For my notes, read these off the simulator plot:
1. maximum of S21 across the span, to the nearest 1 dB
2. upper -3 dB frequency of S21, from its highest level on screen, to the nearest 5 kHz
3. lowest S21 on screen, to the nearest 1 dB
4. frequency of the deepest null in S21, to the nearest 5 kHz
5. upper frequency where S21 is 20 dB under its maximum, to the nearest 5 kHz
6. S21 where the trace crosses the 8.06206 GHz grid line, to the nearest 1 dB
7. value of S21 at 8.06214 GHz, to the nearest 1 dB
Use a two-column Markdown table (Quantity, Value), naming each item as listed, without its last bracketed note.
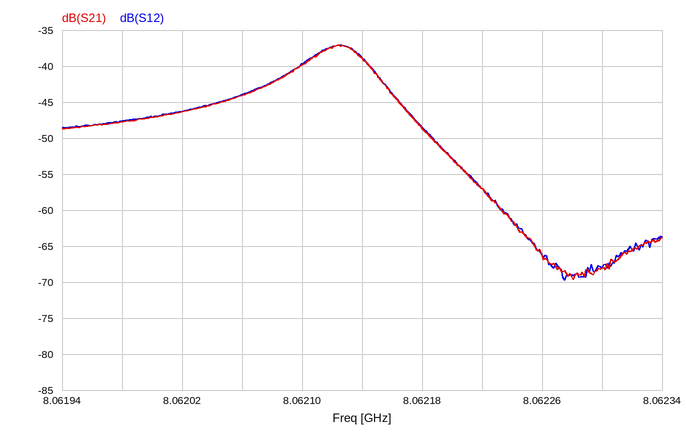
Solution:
| Quantity | Value |
|---|---|
| maximum of S21 across the span, to the nearest 1 dB | -37 dB |
| upper -3 dB frequency of S21, from its highest level on screen, to the nearest 5 kHz | 8.062145 GHz |
| lowest S21 on screen, to the nearest 1 dB | -70 dB |
| frequency of the deepest null in S21, to the nearest 5 kHz | 8.062280 GHz |
| upper frequency where S21 is 20 dB under its maximum, to the nearest 5 kHz | 8.062220 GHz |
| S21 where the trace crosses the 8.06206 GHz grid line, to the nearest 1 dB | -44 dB |
| value of S21 at 8.06214 GHz, to the nearest 1 dB | -39 dB |
